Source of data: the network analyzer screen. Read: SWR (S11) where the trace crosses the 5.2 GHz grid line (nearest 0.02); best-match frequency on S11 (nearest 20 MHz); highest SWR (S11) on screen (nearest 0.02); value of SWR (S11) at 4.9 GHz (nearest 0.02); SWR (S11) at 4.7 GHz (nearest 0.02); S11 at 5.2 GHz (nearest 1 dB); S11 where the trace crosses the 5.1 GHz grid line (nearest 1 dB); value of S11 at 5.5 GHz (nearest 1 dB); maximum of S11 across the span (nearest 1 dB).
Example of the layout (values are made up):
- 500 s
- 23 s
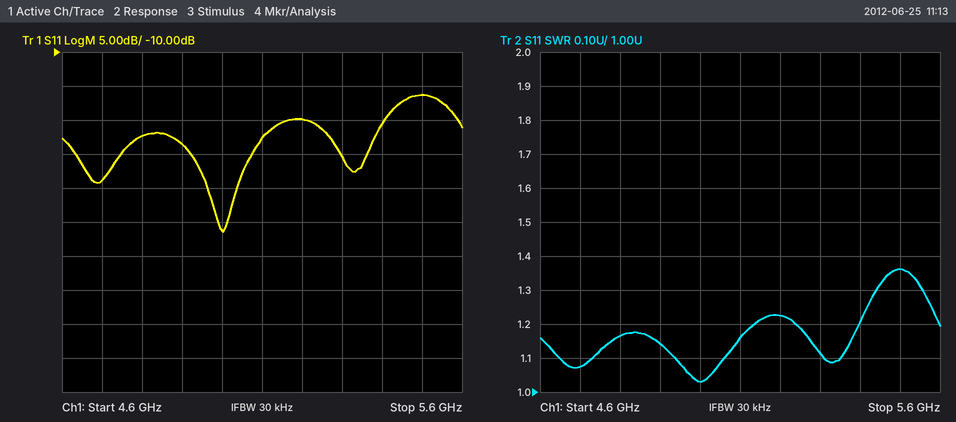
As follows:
- 1.22
- 5.00 GHz
- 1.36
- 1.14
- 1.08
- -20 dB
- -23 dB
- -16 dB
- -16 dB
